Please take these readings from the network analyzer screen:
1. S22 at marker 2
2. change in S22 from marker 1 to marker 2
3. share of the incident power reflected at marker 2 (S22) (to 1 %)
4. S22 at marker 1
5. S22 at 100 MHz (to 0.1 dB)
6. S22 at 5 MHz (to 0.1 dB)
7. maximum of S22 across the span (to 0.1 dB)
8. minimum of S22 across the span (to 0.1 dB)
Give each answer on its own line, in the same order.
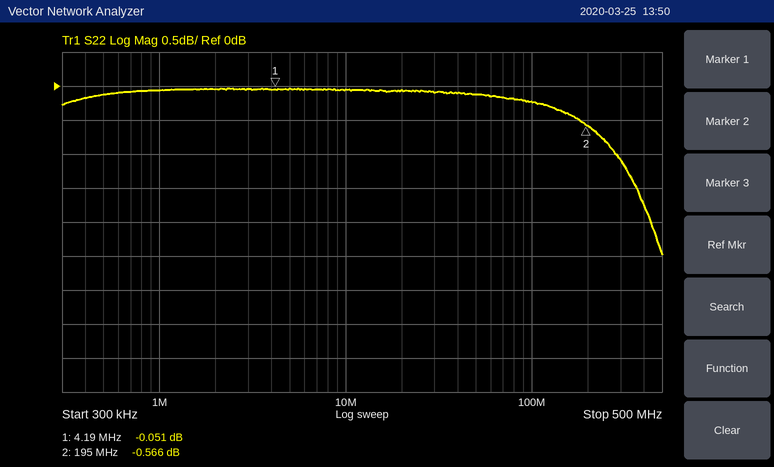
-0.566 dB
-0.515 dB
88 %
-0.051 dB
-0.2 dB
0.0 dB
0.0 dB
-2.5 dB
